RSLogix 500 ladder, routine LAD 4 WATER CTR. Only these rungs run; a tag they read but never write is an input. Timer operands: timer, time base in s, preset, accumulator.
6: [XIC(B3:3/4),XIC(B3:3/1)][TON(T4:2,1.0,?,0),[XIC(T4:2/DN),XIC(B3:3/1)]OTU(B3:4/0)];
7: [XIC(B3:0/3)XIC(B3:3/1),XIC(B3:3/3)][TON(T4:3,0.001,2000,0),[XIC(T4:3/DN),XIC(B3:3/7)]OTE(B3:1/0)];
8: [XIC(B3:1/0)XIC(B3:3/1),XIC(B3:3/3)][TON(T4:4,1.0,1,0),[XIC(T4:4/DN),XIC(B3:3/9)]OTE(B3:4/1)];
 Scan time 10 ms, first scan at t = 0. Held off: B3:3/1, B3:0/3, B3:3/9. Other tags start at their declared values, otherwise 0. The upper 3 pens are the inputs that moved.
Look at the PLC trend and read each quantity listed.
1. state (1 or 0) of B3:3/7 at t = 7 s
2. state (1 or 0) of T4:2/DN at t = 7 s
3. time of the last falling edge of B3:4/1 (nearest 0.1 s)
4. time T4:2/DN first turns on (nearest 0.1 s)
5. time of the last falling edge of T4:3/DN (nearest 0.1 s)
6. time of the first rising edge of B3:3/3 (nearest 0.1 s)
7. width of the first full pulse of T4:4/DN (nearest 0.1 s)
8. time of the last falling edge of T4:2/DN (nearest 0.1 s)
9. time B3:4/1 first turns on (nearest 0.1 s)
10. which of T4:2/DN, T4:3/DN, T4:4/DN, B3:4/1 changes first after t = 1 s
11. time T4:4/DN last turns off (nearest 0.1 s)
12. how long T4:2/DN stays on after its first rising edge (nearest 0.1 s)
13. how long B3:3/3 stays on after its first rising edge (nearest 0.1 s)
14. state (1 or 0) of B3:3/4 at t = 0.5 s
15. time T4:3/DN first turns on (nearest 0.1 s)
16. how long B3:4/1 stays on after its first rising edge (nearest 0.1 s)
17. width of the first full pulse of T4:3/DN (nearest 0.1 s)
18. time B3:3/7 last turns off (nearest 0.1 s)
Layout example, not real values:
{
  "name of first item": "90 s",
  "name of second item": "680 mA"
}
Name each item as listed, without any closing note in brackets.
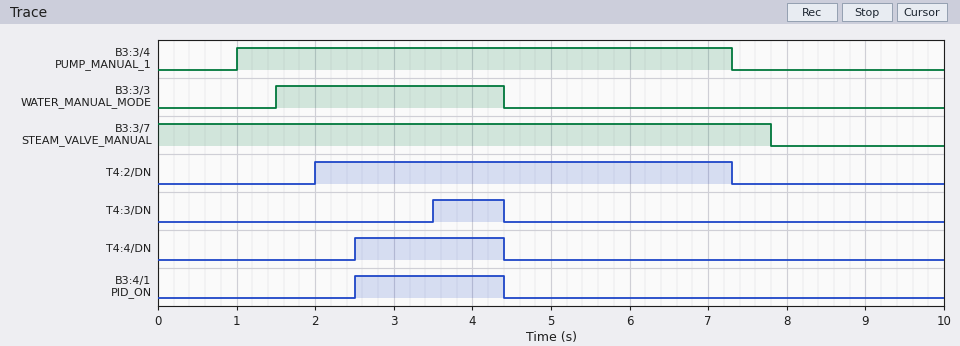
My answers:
{
  "state (1 or 0) of B3:3/7 at t = 7 s": "1",
  "state (1 or 0) of T4:2/DN at t = 7 s": "1",
  "time of the last falling edge of B3:4/1": "4.4 s",
  "time T4:2/DN first turns on": "2.0 s",
  "time of the last falling edge of T4:3/DN": "4.4 s",
  "time of the first rising edge of B3:3/3": "1.5 s",
  "width of the first full pulse of T4:4/DN": "1.9 s",
  "time of the last falling edge of T4:2/DN": "7.3 s",
  "time B3:4/1 first turns on": "2.5 s",
  "which of T4:2/DN, T4:3/DN, T4:4/DN, B3:4/1 changes first after t = 1 s": "T4:2/DN",
  "time T4:4/DN last turns off": "4.4 s",
  "how long T4:2/DN stays on after its first rising edge": "5.3 s",
  "how long B3:3/3 stays on after its first rising edge": "2.9 s",
  "state (1 or 0) of B3:3/4 at t = 0.5 s": "0",
  "time T4:3/DN first turns on": "3.5 s",
  "how long B3:4/1 stays on after its first rising edge": "1.9 s",
  "width of the first full pulse of T4:3/DN": "0.9 s",
  "time B3:3/7 last turns off": "7.8 s"
}
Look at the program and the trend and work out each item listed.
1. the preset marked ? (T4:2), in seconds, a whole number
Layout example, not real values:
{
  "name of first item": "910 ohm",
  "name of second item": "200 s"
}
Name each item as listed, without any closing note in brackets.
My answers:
{
  "the preset marked ? (T4:2), in seconds, a whole number": "1 s"
}
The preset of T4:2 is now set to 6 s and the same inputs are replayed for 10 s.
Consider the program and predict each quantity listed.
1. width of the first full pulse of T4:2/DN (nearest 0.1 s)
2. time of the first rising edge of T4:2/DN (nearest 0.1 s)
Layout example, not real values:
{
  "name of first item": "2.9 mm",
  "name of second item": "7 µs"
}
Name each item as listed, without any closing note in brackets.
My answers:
{
  "width of the first full pulse of T4:2/DN": "0.3 s",
  "time of the first rising edge of T4:2/DN": "7.0 s"
}
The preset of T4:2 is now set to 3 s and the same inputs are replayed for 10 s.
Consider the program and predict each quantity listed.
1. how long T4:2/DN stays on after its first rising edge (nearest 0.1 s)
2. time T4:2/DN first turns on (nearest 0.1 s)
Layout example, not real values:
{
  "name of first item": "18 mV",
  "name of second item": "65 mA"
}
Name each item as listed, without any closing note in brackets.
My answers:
{
  "how long T4:2/DN stays on after its first rising edge": "3.3 s",
  "time T4:2/DN first turns on": "4.0 s"
}
